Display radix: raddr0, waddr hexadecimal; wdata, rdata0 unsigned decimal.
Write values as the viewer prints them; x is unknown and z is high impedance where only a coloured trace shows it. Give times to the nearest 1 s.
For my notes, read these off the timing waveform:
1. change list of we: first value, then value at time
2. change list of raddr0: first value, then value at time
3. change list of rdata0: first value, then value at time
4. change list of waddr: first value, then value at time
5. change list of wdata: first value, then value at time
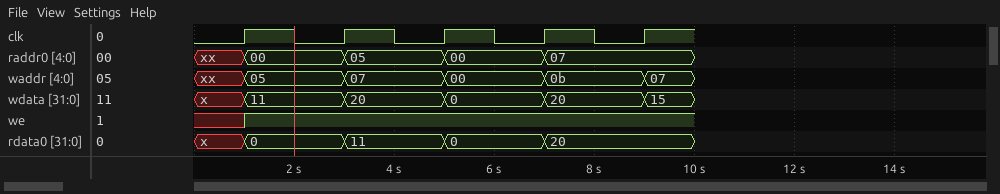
x, 1 at 1 s
xx, 00 at 1 s, 05 at 3 s, 00 at 5 s, 07 at 7 s
x, 0 at 1 s, 11 at 3 s, 0 at 5 s, 20 at 7 s
xx, 05 at 1 s, 07 at 3 s, 00 at 5 s, 0b at 7 s, 07 at 9 s
x, 11 at 1 s, 20 at 3 s, 0 at 5 s, 20 at 7 s, 15 at 9 s
